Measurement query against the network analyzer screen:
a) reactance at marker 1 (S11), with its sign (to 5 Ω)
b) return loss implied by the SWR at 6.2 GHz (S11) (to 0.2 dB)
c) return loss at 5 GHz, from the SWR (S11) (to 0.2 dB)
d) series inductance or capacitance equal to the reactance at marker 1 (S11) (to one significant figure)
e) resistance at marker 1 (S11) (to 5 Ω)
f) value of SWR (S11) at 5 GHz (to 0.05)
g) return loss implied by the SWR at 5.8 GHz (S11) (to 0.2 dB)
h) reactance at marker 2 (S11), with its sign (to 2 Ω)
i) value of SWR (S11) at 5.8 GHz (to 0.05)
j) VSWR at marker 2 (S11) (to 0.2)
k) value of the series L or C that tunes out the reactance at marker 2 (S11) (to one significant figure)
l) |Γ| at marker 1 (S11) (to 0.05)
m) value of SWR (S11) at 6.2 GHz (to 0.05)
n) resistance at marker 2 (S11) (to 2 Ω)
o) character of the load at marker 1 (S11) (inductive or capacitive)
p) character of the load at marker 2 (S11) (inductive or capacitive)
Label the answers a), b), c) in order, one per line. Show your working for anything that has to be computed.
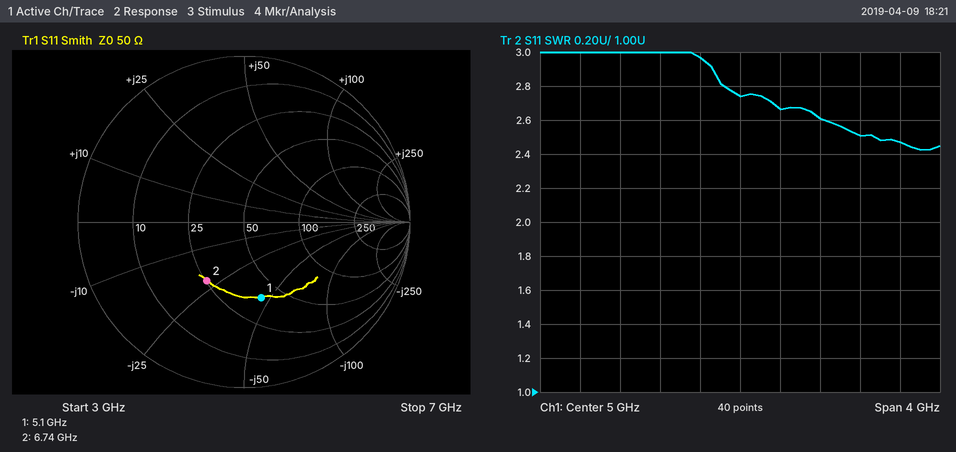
a) -45 Ω
b) −20 log10((2.5 − 1)/(2.5 + 1)) ≈ 7.4 dB
c) −20 log10((2.75 − 1)/(2.75 + 1)) ≈ 6.6 dB
d) C = 1/(2π × 5.1 GHz × 45 Ω) ≈ 693 fF, so 700 fF to one significant figure
e) 40 Ω
f) 2.75
g) −20 log10((2.6 − 1)/(2.6 + 1)) ≈ 7.0 dB
h) -22 Ω
i) 2.60
j) 2.4
k) L = 22 Ω/(2π × 6.74 GHz) ≈ 519 pH, so 500 pH to one significant figure
l) 0.45
m) 2.50
n) 26 Ω
o) capacitive
p) capacitive
